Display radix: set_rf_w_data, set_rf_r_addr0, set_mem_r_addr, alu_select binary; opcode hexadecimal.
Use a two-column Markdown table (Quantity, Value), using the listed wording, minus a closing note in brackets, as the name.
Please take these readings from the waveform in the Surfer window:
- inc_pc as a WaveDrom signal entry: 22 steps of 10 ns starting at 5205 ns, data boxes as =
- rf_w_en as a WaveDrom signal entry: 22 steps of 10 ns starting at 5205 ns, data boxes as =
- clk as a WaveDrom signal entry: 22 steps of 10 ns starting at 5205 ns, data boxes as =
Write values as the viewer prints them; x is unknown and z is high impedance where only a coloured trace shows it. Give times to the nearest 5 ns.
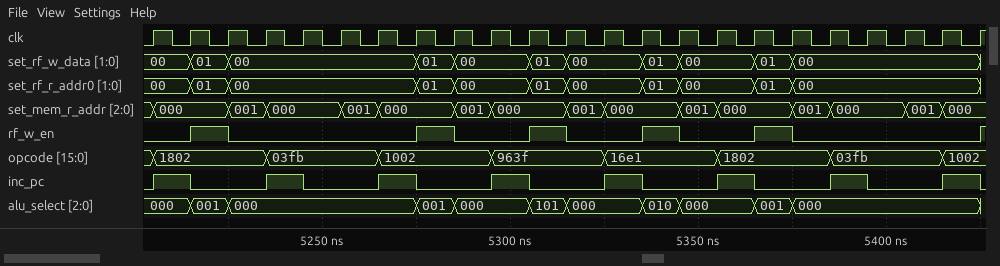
| Quantity | Value |
|---|---|
| inc_pc as a WaveDrom signal entry: 22 steps of 10 ns starting at 5205 ns, data boxes as = | {name: 'inc_pc', wave: '10.10.10.10.10.10.10.1'} |
| rf_w_en as a WaveDrom signal entry: 22 steps of 10 ns starting at 5205 ns, data boxes as = | {name: 'rf_w_en', wave: '010....10.10.10.10....'} |
| clk as a WaveDrom signal entry: 22 steps of 10 ns starting at 5205 ns, data boxes as = | {name: 'clk', wave: 'p.....................'} |
